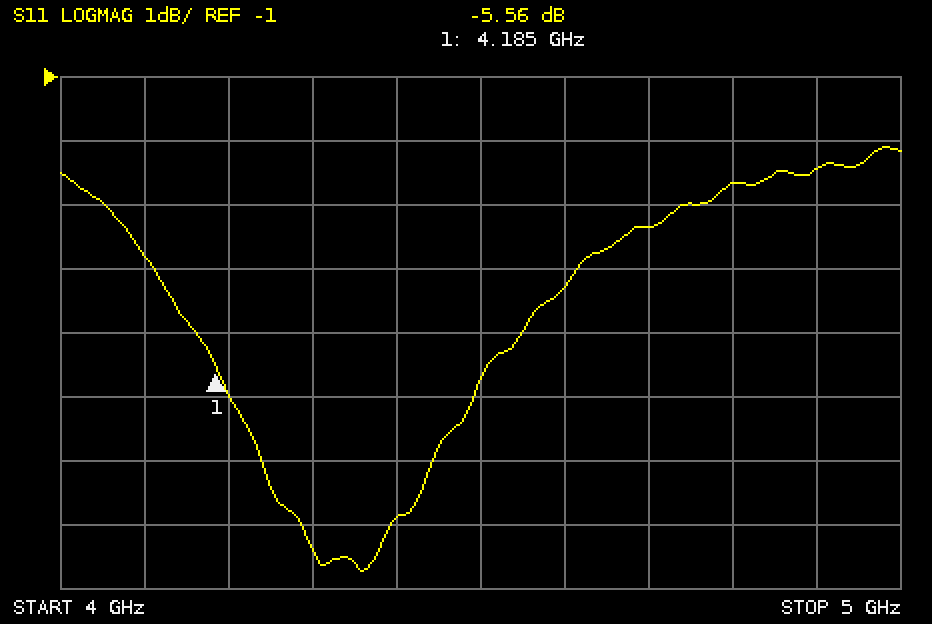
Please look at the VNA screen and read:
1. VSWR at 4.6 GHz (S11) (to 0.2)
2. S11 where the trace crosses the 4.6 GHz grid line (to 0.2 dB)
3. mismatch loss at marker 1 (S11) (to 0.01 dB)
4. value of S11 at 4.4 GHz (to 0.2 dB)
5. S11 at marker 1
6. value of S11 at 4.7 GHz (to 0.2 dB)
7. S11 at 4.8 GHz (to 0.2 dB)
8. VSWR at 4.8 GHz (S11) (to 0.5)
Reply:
4.2
-4.2 dB
1.41 dB
-7.8 dB
-5.56 dB
-3.4 dB
-2.6 dB
6.5
